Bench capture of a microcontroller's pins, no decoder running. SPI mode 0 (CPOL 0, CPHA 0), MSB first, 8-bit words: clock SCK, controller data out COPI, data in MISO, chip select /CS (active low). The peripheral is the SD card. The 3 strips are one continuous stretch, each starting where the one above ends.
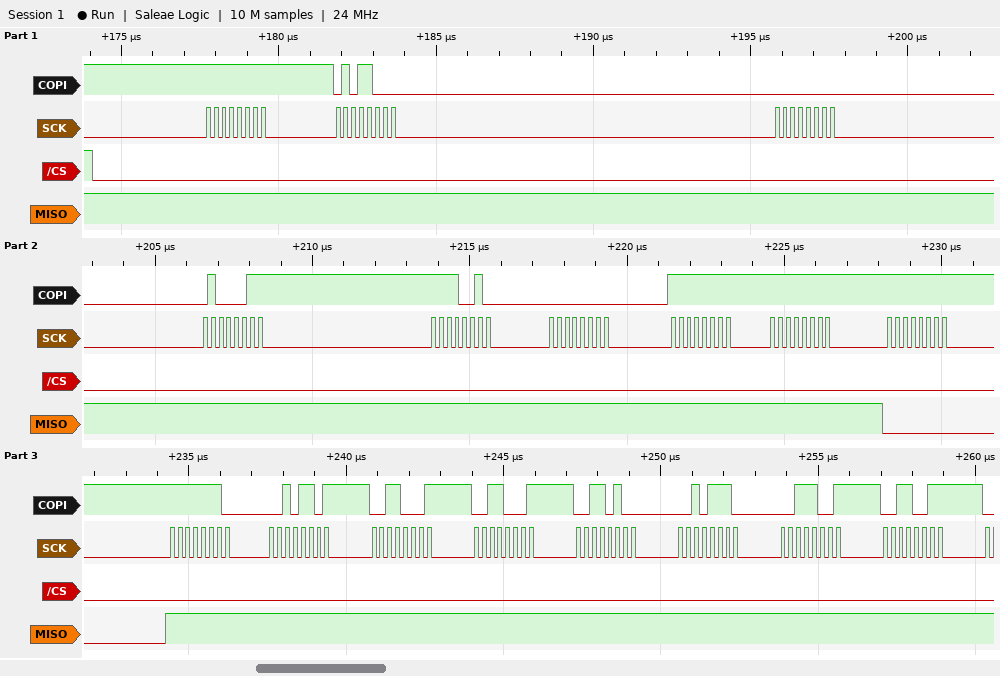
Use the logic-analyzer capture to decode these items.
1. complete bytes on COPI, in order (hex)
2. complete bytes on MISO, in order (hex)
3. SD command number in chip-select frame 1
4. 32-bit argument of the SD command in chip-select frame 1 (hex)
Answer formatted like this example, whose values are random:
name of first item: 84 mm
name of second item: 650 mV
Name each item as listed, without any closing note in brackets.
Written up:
complete bytes on COPI, in order: FF 58 00 43 F2 00 FF FF FF FE 2D 31 31 34 2E 39 33
complete bytes on MISO, in order: FF FF FF FF FF FF FF FF 00 FF FF FF FF FF FF FF FF
SD command number in chip-select frame 1: CMD24
32-bit argument of the SD command in chip-select frame 1: 0x0043F200
